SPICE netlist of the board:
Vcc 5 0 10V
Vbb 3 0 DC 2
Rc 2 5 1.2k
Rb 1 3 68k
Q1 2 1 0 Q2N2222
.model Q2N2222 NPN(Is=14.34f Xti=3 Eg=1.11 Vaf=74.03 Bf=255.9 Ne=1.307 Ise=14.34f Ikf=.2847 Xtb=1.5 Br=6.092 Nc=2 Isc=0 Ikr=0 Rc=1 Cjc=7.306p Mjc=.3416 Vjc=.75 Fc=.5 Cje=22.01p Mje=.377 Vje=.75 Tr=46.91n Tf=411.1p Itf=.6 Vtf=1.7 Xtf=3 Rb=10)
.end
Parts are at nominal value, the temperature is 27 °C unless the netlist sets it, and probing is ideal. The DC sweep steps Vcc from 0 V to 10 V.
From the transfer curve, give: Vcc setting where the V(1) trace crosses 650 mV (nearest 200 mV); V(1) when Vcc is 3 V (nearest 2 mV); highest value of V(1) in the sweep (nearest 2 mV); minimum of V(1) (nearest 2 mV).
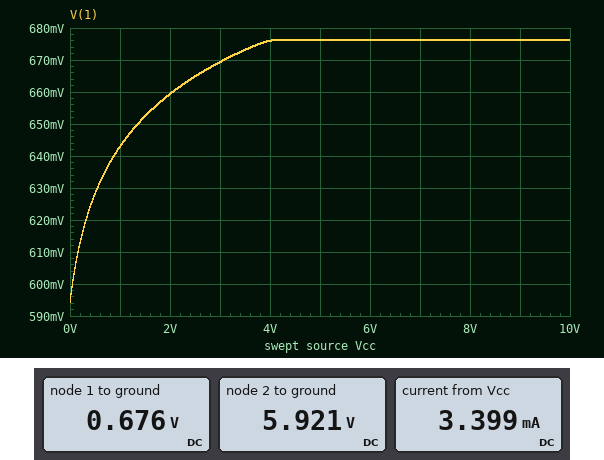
1.4 V
670 mV
676 mV
594 mV
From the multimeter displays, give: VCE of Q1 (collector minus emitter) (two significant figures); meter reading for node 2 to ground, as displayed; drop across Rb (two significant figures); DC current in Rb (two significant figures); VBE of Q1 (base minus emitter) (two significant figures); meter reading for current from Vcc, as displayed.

5.9 V
5.921 V
1.3 V
19 µA
680 mV
3.399 mA
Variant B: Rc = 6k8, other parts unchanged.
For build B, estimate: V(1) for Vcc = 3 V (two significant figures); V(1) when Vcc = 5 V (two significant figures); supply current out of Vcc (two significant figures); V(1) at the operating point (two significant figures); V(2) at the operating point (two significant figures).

630 mV
640 mV
1.5 mA
660 mV
86 mV
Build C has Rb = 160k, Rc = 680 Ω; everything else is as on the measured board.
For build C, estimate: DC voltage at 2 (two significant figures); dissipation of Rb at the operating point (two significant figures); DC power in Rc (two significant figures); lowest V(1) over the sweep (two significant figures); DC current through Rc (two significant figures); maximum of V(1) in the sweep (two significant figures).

9.0 V
11 µW
1.4 mW
570 mV
1.4 mA
650 mV
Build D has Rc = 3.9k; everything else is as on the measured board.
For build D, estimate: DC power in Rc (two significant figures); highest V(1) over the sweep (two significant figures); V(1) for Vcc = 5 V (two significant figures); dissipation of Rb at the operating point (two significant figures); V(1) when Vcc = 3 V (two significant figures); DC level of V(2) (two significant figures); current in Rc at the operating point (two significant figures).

25 mW
670 mV
650 mV
26 µW
640 mV
130 mV
2.5 mA
